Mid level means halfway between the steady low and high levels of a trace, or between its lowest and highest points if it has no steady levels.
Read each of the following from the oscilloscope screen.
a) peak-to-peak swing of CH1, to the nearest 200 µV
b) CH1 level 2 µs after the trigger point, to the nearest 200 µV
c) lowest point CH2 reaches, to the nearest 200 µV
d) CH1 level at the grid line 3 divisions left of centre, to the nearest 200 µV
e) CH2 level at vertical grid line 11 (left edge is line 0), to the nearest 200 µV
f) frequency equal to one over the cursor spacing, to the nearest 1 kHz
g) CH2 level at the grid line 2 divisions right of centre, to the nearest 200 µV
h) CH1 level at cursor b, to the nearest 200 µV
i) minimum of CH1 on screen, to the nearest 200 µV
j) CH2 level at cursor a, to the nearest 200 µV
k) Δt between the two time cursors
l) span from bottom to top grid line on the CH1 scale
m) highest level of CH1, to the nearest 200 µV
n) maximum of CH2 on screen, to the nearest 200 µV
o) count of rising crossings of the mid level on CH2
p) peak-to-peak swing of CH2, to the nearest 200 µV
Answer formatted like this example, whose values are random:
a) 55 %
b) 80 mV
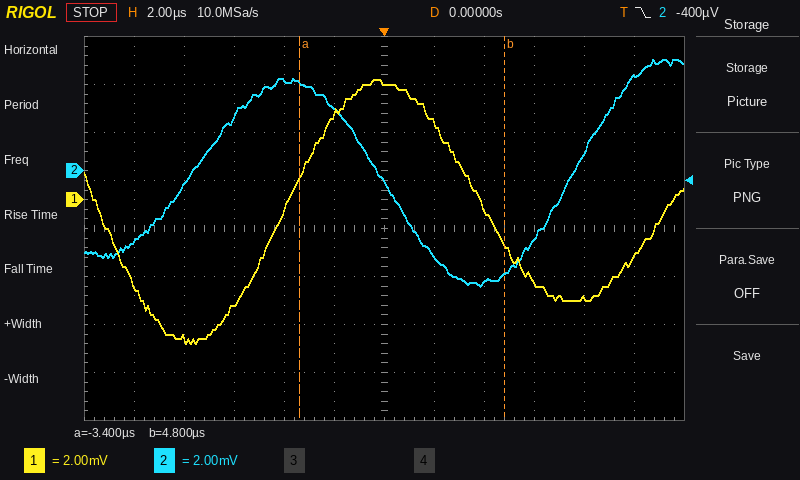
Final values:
a) 11.0 mV
b) 3.2 mV
c) -4.8 mV
d) -4.4 mV
e) 4.0 mV
f) 122 kHz
g) -4.6 mV
h) -1.8 mV
i) -6.0 mV
j) 3.6 mV
k) 8.2 µs
l) 16 mV
m) 5.0 mV
n) 4.6 mV
o) 2
p) 9.4 mV
